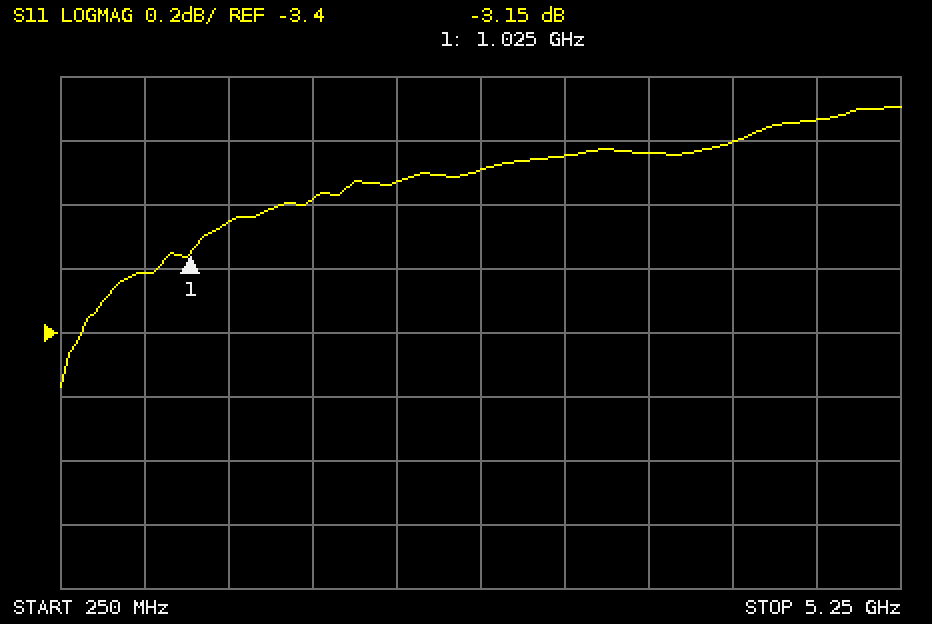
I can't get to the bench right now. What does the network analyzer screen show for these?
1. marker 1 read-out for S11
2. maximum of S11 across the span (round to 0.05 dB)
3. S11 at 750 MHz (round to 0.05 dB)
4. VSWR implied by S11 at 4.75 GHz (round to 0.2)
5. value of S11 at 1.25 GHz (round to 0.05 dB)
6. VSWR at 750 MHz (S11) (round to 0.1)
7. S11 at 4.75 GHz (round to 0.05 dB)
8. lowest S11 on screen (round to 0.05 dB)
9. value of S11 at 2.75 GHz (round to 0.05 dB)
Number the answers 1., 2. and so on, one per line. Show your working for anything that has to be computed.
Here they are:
1. -3.15 dB
2. -2.70 dB
3. -3.20 dB
4. |Γ| = 10^(-2.75/20) = 0.7286; VSWR = (1 + 0.7286)/(1 − 0.7286) ≈ 6.4
5. -3.05 dB
6. |Γ| = 10^(-3.2/20) = 0.6918; VSWR = (1 + 0.6918)/(1 − 0.6918) ≈ 5.5
7. -2.75 dB
8. -3.55 dB
9. -2.90 dB
